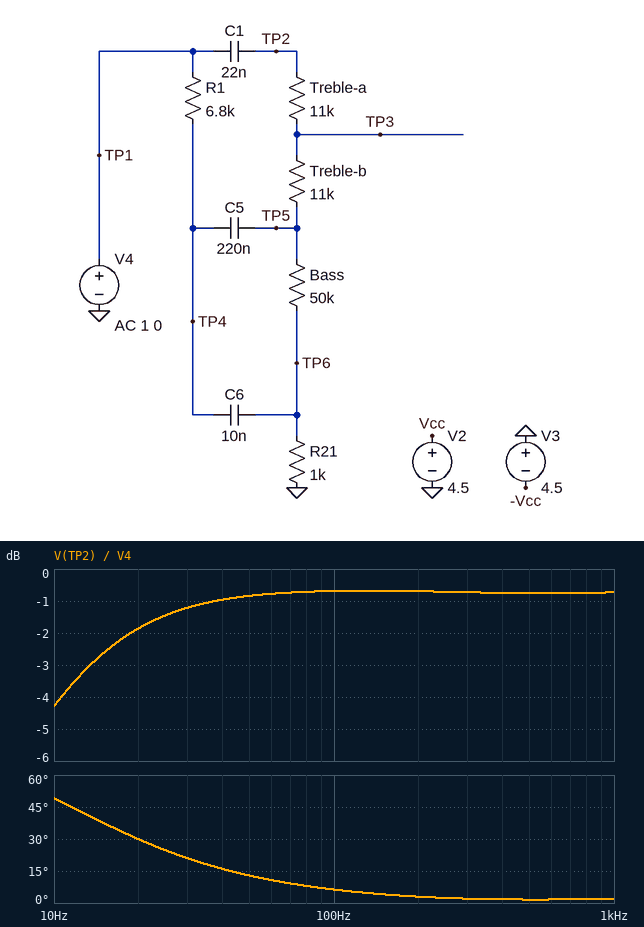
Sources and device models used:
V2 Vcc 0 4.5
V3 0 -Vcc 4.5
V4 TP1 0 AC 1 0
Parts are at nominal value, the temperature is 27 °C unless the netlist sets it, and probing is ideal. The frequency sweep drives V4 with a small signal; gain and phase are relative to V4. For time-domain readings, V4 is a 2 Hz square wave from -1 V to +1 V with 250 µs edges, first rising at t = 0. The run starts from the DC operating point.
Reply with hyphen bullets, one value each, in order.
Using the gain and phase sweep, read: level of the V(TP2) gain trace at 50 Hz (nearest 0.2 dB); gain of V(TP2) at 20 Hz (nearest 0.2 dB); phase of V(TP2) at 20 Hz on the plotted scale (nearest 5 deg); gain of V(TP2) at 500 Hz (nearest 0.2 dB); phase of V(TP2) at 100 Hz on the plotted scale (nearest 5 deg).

- -0.8 dB
- -1.8 dB
- 30 deg
- -0.8 dB
- 5 deg
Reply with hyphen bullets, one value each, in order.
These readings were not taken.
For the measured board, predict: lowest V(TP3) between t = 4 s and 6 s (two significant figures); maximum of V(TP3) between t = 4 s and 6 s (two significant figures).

- -1.8 V
- 1.8 V
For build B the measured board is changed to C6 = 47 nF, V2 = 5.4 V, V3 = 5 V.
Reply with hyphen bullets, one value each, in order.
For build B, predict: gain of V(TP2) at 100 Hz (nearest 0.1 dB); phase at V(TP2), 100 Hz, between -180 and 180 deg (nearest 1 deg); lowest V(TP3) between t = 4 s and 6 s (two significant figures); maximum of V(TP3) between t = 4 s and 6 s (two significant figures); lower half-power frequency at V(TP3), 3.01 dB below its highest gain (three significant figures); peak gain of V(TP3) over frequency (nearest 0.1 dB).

- -1.2 dB
- 1 deg
- -1.6 V
- 1.6 V
- 10.8 Hz
- -1.1 dB
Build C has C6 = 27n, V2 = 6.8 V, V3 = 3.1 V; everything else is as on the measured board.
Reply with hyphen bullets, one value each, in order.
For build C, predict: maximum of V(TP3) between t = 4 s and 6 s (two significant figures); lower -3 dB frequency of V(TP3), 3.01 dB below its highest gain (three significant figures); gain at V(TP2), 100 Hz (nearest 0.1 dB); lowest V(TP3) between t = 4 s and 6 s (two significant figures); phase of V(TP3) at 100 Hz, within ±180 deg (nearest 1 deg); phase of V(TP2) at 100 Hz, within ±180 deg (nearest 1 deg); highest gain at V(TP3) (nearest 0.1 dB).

- 1.7 V
- 11.1 Hz
- -0.9 dB
- -1.7 V
- 3 deg
- 4 deg
- -1.0 dB
